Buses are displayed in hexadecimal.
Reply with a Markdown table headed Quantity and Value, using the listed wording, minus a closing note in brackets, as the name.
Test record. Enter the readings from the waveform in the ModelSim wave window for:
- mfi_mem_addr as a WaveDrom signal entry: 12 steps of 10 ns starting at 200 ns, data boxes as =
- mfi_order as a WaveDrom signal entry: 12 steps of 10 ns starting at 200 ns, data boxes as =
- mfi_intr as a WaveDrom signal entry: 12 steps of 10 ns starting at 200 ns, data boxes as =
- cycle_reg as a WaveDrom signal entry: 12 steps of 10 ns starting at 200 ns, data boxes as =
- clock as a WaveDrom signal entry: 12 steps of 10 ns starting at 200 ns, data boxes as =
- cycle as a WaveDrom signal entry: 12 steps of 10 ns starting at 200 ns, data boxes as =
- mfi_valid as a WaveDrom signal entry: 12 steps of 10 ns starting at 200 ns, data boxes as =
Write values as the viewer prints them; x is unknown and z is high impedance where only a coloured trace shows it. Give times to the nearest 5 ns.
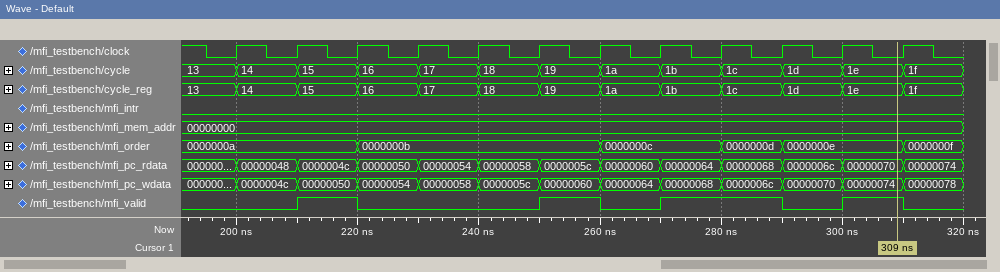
| Quantity | Value |
|---|---|
| mfi_mem_addr as a WaveDrom signal entry: 12 steps of 10 ns starting at 200 ns, data boxes as = | {name: 'mfi_mem_addr', wave: '=...........', data: '00000000'} |
| mfi_order as a WaveDrom signal entry: 12 steps of 10 ns starting at 200 ns, data boxes as = | {name: 'mfi_order', wave: '=.=...=.==.=', data: '0000000a 0000000b 0000000c 0000000d 0000000e 0000000f'} |
| mfi_intr as a WaveDrom signal entry: 12 steps of 10 ns starting at 200 ns, data boxes as = | {name: 'mfi_intr', wave: '0...........'} |
| cycle_reg as a WaveDrom signal entry: 12 steps of 10 ns starting at 200 ns, data boxes as = | {name: 'cycle_reg', wave: '============', data: '14 15 16 17 18 19 1a 1b 1c 1d 1e 1f'} |
| clock as a WaveDrom signal entry: 12 steps of 10 ns starting at 200 ns, data boxes as = | {name: 'clock', wave: 'p...........'} |
| cycle as a WaveDrom signal entry: 12 steps of 10 ns starting at 200 ns, data boxes as = | {name: 'cycle', wave: '============', data: '14 15 16 17 18 19 1a 1b 1c 1d 1e 1f'} |
| mfi_valid as a WaveDrom signal entry: 12 steps of 10 ns starting at 200 ns, data boxes as = | {name: 'mfi_valid', wave: '010..101.010'} |
